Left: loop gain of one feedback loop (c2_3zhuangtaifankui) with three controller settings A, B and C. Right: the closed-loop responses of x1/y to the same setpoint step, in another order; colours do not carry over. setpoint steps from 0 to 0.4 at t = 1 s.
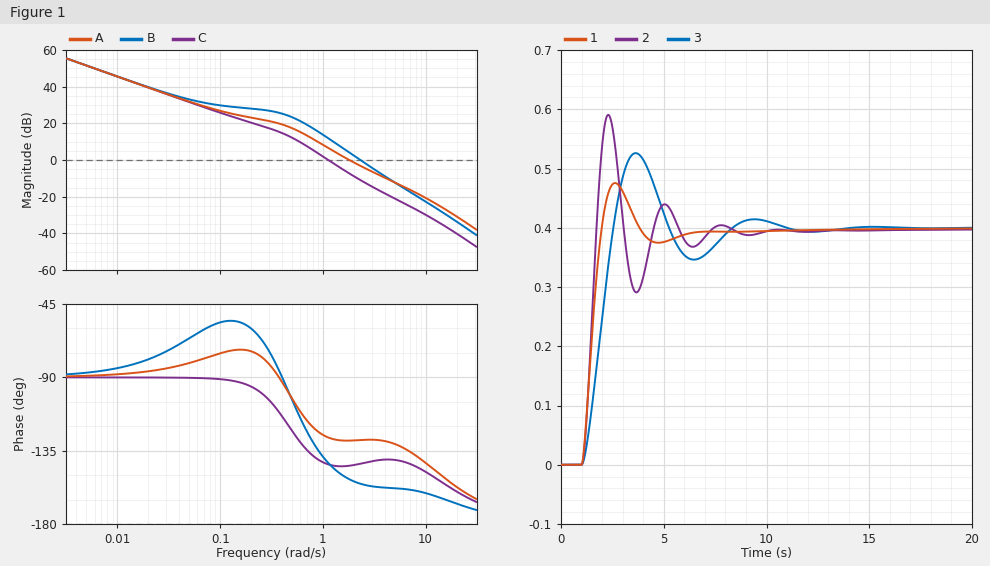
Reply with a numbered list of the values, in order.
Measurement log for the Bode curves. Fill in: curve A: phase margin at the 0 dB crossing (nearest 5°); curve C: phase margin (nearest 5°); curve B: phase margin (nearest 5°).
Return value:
1. 50°
2. 35°
3. 25°
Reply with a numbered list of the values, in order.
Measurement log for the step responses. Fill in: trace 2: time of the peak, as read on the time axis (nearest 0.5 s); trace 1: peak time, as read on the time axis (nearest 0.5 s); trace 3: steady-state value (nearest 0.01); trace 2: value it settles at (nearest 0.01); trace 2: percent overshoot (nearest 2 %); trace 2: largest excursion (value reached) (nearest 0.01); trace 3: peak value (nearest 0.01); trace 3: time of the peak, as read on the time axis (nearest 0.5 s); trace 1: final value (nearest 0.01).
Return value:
1. 2.5 s
2. 2.5 s
3. 0.40
4. 0.40
5. 48 %
6. 0.59
7. 0.53
8. 3.5 s
9. 0.40
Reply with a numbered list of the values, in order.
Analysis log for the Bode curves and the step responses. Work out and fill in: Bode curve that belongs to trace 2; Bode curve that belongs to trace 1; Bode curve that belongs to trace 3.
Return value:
1. B
2. A
3. C
